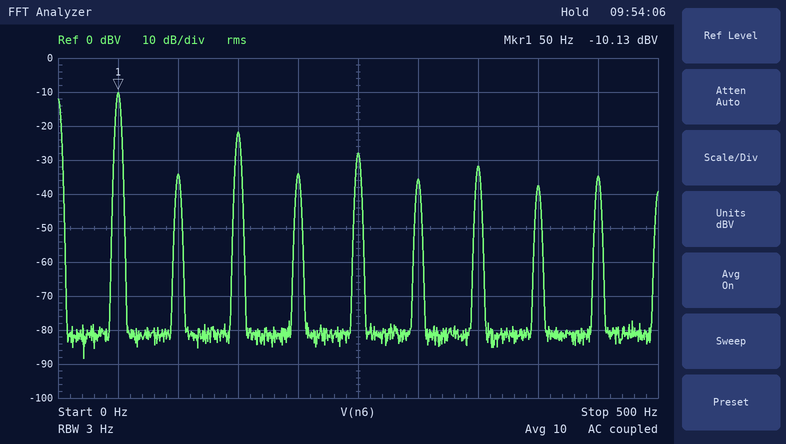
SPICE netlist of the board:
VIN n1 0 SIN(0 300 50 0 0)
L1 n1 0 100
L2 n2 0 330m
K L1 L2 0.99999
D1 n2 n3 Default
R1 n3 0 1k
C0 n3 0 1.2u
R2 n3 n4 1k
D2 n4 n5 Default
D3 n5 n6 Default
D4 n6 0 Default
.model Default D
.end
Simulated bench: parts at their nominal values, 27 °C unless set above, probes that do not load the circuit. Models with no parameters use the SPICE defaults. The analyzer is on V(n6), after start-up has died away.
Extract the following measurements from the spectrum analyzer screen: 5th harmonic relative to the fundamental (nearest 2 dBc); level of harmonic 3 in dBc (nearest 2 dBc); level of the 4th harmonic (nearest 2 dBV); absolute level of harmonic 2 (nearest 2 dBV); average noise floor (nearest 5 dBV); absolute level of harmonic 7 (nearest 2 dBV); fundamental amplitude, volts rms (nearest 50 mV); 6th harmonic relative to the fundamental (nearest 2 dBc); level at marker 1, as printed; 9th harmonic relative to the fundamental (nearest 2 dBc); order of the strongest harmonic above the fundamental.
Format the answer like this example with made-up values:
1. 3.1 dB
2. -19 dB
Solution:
1. -18 dBc
2. -12 dBc
3. -34 dBV
4. -34 dBV
5. -80 dBV
6. -32 dBV
7. 300 mV
8. -26 dBc
9. -10.13 dBV
10. -24 dBc
11. 3
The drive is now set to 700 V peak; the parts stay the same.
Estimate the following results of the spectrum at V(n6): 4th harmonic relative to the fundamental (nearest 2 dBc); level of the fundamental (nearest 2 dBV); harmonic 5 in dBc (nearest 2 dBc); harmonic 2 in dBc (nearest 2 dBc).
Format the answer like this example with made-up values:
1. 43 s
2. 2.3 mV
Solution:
1. -18 dBc
2. -10 dBV
3. -20 dBc
4. -16 dBc
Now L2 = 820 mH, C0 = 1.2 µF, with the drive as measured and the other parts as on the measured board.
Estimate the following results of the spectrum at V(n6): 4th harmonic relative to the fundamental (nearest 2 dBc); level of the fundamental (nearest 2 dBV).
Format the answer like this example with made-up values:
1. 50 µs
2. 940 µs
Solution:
1. -20 dBc
2. -10 dBV
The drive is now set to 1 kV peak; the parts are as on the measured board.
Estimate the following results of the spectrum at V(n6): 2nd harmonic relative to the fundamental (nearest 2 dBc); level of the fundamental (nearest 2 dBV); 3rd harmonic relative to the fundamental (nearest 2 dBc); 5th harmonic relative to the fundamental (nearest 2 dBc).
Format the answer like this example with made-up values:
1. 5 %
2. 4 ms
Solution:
1. -14 dBc
2. -10 dBV
3. -14 dBc
4. -20 dBc
